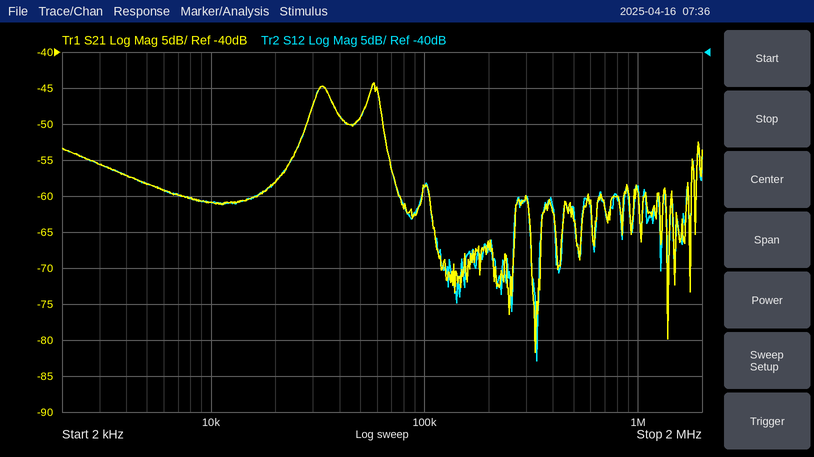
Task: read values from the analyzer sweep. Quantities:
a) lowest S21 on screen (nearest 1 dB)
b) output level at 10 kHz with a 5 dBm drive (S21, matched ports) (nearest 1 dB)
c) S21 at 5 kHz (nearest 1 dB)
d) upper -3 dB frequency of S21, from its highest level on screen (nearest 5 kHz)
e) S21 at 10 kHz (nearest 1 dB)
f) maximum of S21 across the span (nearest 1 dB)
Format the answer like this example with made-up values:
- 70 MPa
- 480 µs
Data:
- -82 dB
- -56 dBm
- -58 dB
- 60 kHz
- -61 dB
- -44 dB
